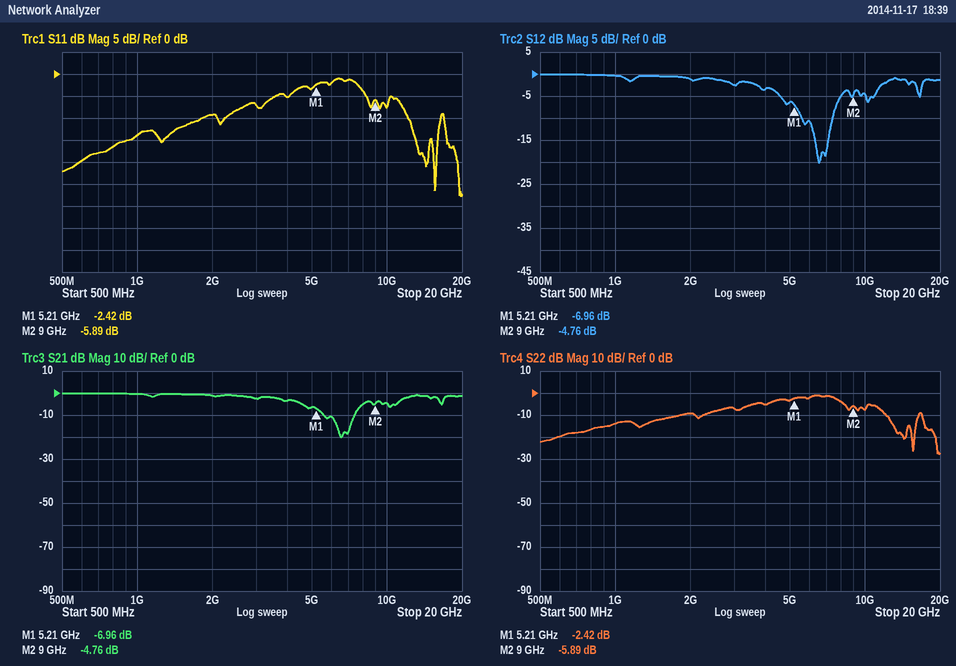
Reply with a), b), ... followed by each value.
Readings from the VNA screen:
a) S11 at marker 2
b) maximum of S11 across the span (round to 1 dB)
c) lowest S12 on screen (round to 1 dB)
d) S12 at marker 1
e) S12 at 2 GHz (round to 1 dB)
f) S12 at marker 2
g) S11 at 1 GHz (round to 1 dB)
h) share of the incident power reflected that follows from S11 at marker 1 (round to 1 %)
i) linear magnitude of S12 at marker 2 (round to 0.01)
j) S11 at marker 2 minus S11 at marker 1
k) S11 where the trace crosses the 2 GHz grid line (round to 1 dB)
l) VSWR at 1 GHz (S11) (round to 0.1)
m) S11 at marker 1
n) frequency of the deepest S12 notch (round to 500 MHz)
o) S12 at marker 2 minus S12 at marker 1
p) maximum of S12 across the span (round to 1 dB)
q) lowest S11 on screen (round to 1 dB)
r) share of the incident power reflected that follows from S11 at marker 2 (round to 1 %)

a) -5.89 dB
b) -1 dB
c) -20 dB
d) -6.96 dB
e) -1 dB
f) -4.76 dB
g) -14 dB
h) 57 %
i) 0.58
j) -3.47 dB
k) -9 dB
l) 1.5
m) -2.42 dB
n) 6.5 GHz
o) 2.20 dB
p) 0 dB
q) -28 dB
r) 26 %
